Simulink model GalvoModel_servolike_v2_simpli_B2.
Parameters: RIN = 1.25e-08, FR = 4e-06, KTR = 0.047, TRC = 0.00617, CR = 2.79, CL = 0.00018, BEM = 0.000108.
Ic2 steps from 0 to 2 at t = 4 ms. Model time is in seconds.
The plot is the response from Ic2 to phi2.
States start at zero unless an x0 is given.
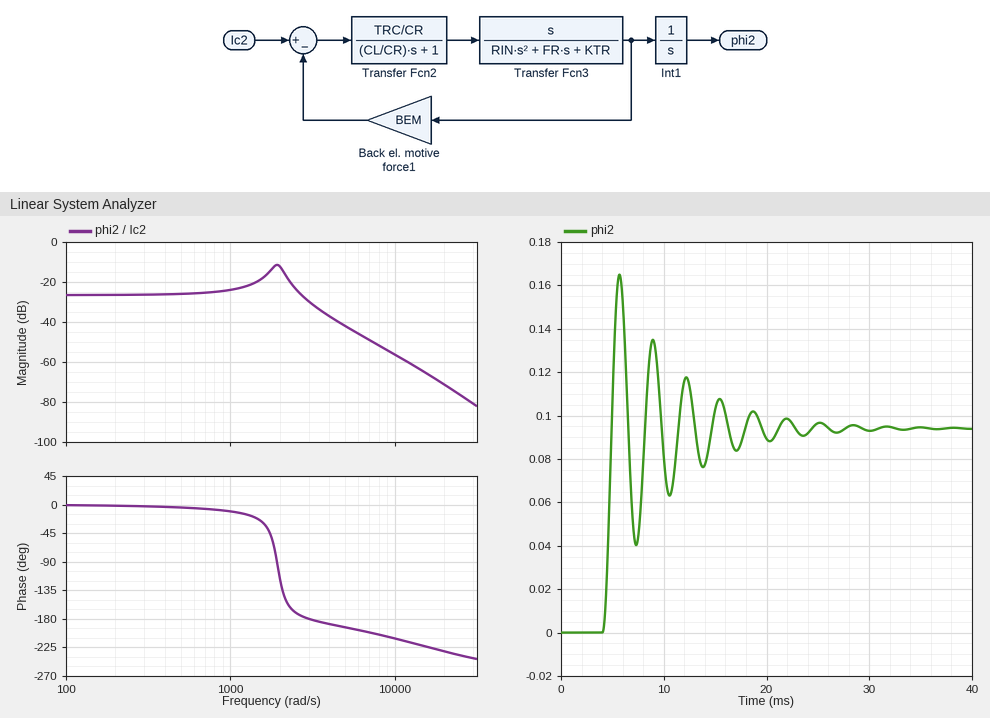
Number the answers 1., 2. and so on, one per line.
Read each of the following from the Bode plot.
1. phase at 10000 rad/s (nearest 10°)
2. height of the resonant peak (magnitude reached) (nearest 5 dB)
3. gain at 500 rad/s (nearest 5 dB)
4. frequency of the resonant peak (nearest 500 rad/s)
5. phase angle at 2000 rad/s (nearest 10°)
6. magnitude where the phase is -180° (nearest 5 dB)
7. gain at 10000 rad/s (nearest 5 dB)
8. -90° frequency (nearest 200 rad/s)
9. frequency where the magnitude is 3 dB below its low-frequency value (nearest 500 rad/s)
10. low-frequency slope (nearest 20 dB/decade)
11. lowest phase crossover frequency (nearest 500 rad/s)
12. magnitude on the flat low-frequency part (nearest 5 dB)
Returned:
1. -210°
2. -10 dB
3. -25 dB
4. 2000 rad/s
5. -120°
6. -30 dB
7. -55 dB
8. 2000 rad/s
9. 3000 rad/s
10. 0 dB/decade
11. 3000 rad/s
12. -25 dB
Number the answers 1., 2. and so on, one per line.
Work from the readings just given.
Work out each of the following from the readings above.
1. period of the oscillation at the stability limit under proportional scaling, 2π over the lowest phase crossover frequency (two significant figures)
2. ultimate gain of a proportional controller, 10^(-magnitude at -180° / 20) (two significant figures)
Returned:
1. 0.0021 s
2. 32
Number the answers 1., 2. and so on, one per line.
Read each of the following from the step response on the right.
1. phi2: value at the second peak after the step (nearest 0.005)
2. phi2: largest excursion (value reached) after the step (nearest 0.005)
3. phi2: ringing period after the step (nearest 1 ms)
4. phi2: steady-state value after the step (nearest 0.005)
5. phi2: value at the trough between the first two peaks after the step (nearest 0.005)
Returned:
1. 0.135
2. 0.165
3. 3 ms
4. 0.095
5. 0.040
